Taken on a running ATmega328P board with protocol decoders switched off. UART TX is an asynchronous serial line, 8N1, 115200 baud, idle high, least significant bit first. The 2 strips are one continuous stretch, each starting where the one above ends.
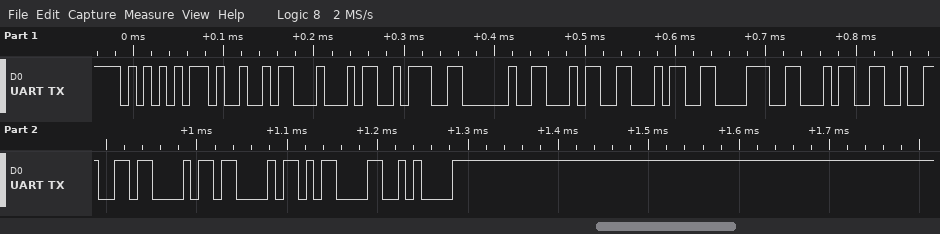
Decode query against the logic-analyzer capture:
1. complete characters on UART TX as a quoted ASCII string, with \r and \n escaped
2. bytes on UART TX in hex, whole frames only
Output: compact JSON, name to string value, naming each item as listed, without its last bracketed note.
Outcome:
{"complete characters on UART TX as a quoted ASCII string, with \\r and \\n escaped": "\"UID: 44842CC\\r\\n\"", "bytes on UART TX in hex, whole frames only": "0x55 0x49 0x44 0x3A 0x20 0x34 0x34 0x38 0x34 0x32 0x43 0x43 0x0D 0x0A"}
